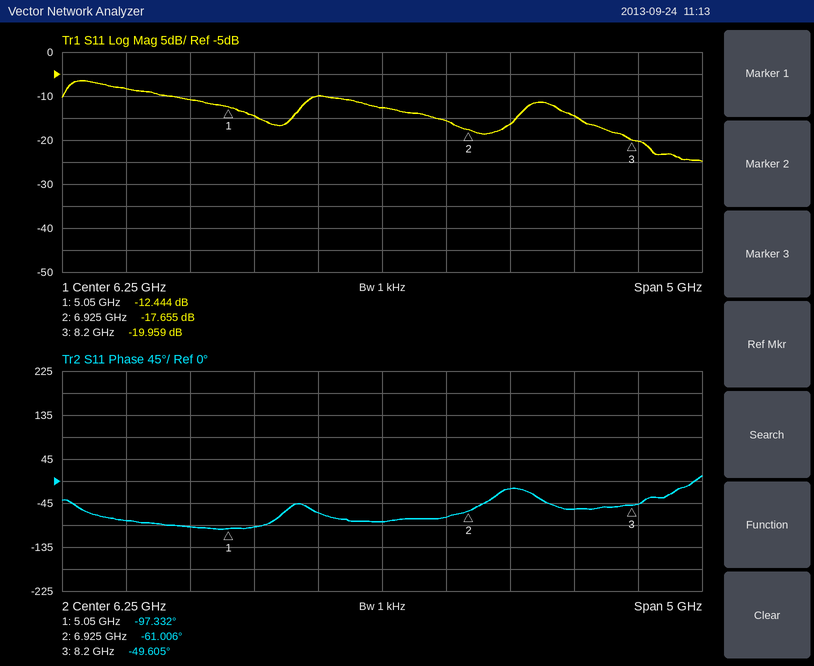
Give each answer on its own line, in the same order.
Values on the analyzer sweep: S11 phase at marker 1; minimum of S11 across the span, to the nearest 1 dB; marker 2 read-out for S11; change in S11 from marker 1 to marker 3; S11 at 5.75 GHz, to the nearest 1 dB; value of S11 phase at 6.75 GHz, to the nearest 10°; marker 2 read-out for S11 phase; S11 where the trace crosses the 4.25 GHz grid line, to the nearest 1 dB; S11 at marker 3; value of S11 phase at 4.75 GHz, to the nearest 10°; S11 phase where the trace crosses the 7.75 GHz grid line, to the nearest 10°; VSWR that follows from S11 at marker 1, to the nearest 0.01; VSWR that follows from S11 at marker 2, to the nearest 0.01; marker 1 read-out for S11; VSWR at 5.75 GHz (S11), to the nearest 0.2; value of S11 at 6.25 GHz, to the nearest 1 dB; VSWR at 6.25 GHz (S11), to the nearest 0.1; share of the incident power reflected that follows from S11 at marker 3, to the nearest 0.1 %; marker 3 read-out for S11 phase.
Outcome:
-97.332°
-25 dB
-17.655 dB
-7.515 dB
-10 dB
-70°
-61.006°
-8 dB
-19.959 dB
-90°
-60°
1.63
1.30
-12.444 dB
2.0
-13 dB
1.6
1.0 %
-49.605°
